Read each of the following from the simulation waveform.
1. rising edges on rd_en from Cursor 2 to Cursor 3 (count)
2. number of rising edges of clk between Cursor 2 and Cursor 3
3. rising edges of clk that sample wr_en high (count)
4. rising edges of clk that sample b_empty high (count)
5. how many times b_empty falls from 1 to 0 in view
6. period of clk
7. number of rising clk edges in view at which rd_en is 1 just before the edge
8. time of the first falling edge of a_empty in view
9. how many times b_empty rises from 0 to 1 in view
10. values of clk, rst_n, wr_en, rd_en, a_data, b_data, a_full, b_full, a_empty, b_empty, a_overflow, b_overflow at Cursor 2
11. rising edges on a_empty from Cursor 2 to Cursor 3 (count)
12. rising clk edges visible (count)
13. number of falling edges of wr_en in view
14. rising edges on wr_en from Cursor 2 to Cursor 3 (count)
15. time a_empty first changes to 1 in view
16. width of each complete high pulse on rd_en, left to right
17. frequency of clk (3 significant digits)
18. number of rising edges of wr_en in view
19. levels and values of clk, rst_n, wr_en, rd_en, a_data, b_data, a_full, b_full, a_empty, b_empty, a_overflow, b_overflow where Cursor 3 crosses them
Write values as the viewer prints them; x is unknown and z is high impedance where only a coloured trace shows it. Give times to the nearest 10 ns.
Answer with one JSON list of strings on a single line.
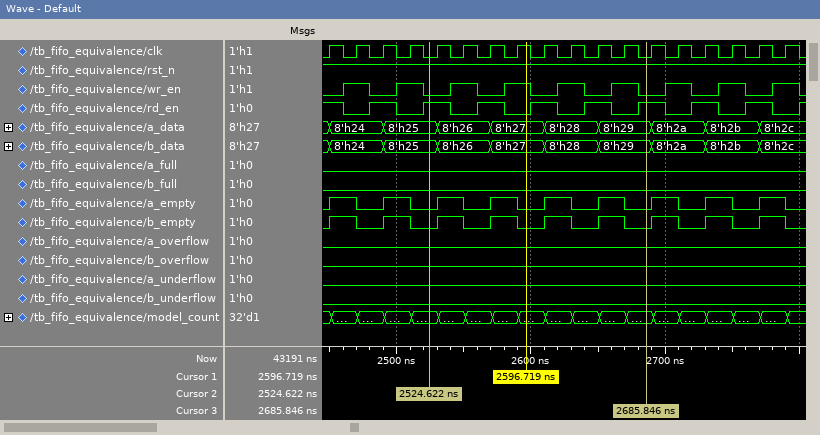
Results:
["4", "8", "9", "9", "9", "20 ns", "9", "2470 ns", "9", "clk=0, rst_n=1, wr_en=0, rd_en=1, a_data=8'h25, b_data=8'h25, a_full=0, b_full=0, a_empty=0, b_empty=0, a_overflow=0, b_overflow=0", "4", "18", "9", "4", "2450 ns", "20 ns, 20 ns, 20 ns, 20 ns, 20 ns, 20 ns, 20 ns, 20 ns", "50.0 MHz", "9", "clk=0, rst_n=1, wr_en=0, rd_en=1, a_data=8'h29, b_data=8'h29, a_full=0, b_full=0, a_empty=0, b_empty=0, a_overflow=0, b_overflow=0"]
